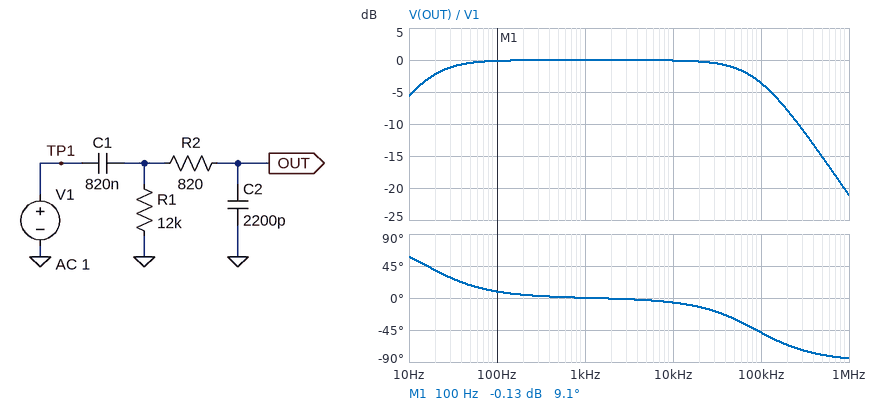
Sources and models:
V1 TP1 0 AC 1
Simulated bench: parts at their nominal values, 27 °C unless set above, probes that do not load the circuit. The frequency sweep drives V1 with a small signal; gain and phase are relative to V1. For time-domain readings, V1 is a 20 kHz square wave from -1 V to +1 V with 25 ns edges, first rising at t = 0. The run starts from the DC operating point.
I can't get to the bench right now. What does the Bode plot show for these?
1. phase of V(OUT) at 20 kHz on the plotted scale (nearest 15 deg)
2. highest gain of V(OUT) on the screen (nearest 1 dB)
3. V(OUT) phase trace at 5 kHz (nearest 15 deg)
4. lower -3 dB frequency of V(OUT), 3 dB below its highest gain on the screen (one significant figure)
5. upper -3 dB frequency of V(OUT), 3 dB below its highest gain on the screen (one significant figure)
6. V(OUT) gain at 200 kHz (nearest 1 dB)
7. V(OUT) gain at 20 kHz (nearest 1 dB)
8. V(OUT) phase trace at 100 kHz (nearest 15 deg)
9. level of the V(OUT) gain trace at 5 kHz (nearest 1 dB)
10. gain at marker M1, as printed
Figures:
-15 deg
0 dB
0 deg
20 Hz
90 kHz
-8 dB
0 dB
-45 deg
0 dB
-0.13 dB
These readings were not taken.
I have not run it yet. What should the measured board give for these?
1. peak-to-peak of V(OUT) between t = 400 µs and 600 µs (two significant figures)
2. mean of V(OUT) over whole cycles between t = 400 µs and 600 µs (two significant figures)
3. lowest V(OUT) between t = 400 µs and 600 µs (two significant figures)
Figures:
2.0 V
950 mV
-59 mV
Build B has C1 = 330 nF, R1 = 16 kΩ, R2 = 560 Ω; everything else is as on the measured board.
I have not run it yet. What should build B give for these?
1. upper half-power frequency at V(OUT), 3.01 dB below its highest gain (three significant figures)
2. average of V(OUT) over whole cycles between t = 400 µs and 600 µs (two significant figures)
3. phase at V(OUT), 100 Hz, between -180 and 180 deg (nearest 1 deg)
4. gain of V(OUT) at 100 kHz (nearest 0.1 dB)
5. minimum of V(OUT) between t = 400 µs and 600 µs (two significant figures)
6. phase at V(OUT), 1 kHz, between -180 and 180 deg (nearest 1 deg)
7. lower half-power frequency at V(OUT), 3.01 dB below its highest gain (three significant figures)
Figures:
130 kHz
910 mV
17 deg
-2.1 dB
-110 mV
1 deg
29.9 Hz
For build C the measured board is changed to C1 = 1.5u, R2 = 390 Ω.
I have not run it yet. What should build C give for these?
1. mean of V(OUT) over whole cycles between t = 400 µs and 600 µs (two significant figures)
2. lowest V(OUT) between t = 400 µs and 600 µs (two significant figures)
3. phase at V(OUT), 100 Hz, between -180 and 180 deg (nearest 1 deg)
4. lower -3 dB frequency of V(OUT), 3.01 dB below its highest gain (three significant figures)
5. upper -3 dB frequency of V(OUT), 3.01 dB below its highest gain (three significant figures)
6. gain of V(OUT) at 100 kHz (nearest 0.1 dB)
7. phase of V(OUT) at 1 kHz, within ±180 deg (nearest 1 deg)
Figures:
970 mV
-33 mV
5 deg
8.83 Hz
186 kHz
-1.1 dB
0 deg
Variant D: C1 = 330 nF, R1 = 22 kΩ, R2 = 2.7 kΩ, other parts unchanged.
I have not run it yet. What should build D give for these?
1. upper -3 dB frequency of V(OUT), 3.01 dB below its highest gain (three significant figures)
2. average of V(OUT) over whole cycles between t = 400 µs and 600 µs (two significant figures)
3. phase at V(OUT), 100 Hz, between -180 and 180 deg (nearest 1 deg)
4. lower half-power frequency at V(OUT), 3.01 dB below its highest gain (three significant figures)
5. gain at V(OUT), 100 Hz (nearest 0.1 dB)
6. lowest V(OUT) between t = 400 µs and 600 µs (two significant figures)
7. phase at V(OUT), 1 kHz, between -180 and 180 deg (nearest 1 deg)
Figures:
27.0 kHz
930 mV
12 deg
21.7 Hz
-0.3 dB
-50 mV
-1 deg
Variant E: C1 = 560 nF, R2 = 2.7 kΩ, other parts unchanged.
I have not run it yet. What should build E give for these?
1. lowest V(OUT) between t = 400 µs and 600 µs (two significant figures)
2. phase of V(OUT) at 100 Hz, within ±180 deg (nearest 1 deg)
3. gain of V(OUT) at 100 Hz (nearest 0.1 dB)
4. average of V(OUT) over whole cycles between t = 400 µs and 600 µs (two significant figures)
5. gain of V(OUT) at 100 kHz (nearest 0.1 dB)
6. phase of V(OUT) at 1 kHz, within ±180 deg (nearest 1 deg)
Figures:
-56 mV
13 deg
-0.3 dB
930 mV
-11.7 dB
-1 deg
